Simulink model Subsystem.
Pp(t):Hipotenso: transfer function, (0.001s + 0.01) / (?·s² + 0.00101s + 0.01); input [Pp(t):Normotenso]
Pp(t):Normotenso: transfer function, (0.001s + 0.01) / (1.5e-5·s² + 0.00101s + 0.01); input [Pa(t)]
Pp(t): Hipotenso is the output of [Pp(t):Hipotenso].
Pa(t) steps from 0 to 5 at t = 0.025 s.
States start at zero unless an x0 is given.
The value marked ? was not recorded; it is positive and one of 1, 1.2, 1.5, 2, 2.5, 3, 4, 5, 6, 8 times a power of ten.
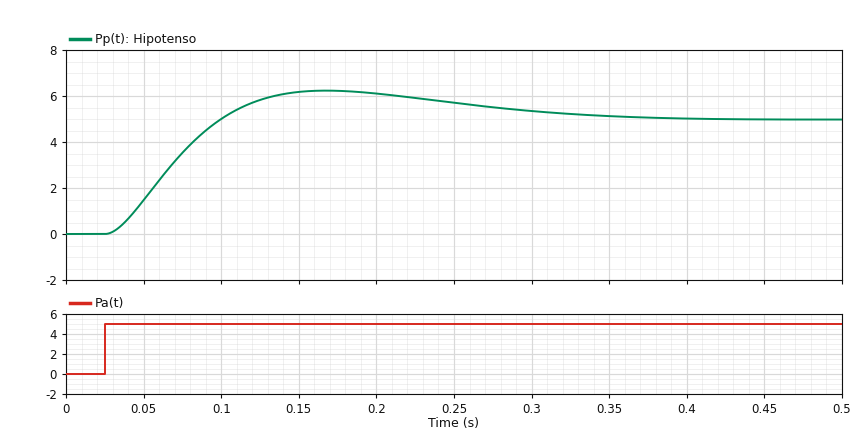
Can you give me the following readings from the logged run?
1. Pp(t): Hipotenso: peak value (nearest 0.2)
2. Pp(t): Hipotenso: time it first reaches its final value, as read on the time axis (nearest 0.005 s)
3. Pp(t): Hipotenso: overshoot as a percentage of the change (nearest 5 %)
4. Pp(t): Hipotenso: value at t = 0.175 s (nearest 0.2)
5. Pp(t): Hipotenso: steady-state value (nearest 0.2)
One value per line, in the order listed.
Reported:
6.2
0.100 s
25 %
6.2
5.0
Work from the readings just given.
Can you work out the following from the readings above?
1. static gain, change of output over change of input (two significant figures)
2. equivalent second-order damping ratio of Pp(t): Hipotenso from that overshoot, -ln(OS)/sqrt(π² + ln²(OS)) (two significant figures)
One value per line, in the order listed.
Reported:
1.0
0.40
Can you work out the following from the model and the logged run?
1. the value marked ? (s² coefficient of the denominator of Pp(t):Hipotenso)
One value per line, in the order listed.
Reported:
4e-05
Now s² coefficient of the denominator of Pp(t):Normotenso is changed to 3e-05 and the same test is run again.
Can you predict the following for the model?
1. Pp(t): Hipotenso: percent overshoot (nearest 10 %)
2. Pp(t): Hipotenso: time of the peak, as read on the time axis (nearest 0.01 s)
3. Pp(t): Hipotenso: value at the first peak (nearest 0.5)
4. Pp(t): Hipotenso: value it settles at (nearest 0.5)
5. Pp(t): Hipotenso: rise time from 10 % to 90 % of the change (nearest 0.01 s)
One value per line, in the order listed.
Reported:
30 %
0.19 s
6.5
5.0
0.06 s
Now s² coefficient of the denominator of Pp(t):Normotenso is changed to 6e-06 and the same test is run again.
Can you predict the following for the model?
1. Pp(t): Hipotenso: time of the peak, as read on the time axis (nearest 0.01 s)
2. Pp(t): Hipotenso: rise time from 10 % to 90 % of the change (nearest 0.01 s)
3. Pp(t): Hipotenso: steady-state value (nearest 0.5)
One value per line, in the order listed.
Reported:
0.16 s
0.05 s
5.0
